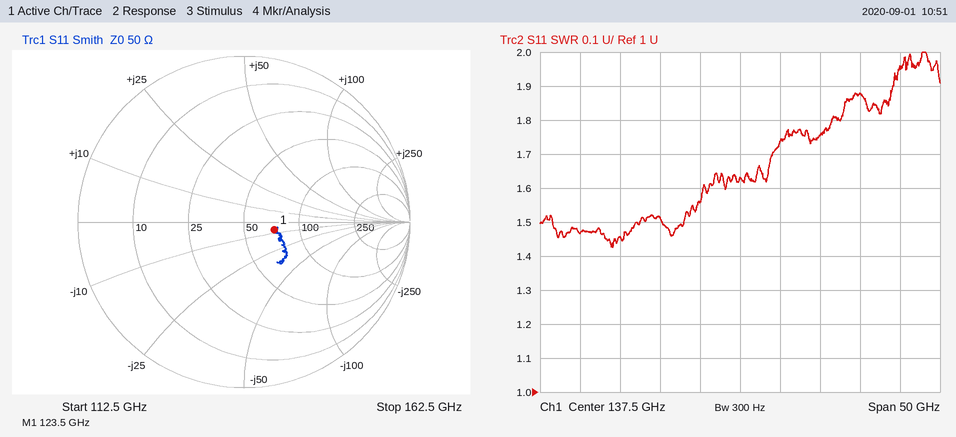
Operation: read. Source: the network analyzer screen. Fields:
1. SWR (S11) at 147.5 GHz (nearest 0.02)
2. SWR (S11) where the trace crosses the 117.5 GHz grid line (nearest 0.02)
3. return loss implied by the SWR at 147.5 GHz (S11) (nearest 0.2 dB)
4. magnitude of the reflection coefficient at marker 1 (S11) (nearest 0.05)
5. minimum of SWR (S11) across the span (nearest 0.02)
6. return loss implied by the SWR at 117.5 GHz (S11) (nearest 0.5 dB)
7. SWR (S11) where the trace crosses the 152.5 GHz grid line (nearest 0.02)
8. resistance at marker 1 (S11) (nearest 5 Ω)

1.76
1.46
11.2 dB
0.20
1.42
14.5 dB
1.88
70 Ω
